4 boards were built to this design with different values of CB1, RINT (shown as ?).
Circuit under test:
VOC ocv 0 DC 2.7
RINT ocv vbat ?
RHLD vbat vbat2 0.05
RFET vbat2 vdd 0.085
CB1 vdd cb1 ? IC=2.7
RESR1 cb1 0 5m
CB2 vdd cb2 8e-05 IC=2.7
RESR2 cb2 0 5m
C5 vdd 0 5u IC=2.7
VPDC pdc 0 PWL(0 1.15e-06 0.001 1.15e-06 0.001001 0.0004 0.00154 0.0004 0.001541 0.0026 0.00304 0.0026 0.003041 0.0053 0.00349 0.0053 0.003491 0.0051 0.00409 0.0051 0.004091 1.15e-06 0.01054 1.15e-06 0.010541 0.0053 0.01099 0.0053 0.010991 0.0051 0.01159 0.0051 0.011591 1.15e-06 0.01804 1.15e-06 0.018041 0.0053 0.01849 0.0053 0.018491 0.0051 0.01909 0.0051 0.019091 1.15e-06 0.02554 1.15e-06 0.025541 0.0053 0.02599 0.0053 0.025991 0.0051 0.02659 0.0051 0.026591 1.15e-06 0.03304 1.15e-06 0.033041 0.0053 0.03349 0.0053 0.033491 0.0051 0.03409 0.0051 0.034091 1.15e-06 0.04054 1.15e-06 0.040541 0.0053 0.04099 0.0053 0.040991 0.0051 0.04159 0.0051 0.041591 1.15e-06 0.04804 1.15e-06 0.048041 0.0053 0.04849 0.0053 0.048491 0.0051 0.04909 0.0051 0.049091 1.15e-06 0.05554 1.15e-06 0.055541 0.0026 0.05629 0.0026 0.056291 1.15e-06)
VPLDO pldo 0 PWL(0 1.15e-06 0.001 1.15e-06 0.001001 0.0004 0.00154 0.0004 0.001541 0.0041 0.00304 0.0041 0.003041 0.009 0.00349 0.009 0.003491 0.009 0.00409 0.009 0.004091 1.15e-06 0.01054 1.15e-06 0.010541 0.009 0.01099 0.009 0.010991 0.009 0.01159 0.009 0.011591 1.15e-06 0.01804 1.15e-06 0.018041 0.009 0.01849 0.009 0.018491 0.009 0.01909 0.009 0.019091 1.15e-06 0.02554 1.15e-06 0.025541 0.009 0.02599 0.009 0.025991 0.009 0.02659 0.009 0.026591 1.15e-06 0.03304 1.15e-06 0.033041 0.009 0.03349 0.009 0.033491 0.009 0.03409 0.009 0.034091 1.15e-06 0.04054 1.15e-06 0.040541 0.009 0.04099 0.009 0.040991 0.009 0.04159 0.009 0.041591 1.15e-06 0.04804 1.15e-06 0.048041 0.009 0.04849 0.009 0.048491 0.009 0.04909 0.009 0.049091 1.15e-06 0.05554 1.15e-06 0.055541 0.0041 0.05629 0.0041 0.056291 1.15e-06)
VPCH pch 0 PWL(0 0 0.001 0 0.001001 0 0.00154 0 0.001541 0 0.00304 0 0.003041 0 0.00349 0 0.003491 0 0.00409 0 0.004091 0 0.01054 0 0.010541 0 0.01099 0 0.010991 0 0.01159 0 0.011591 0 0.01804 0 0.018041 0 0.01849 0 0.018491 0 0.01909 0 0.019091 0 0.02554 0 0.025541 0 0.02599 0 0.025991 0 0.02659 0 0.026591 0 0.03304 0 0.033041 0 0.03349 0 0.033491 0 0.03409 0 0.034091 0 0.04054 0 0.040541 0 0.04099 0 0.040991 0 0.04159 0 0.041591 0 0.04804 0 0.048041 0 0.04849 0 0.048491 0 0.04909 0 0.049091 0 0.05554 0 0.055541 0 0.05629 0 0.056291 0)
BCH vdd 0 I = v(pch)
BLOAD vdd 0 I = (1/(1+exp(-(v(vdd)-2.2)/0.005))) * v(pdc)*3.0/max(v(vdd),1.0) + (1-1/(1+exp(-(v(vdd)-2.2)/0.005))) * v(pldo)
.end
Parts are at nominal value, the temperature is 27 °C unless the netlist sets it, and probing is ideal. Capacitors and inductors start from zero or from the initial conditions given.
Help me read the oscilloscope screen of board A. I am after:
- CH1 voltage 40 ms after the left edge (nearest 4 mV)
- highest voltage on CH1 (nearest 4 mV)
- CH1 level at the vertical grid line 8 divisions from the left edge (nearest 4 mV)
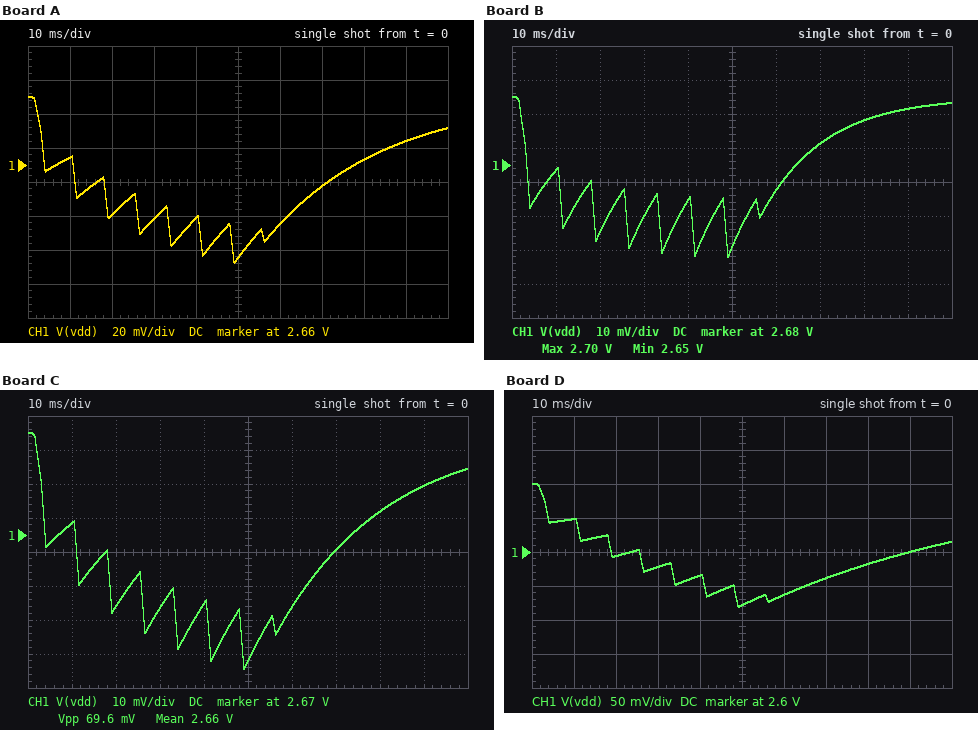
2.628 V
2.700 V
2.664 V
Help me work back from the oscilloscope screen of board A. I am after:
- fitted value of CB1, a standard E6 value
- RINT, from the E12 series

150 µF
120 Ω
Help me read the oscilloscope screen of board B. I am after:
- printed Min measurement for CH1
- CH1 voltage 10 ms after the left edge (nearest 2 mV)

2.65 V
2.678 V
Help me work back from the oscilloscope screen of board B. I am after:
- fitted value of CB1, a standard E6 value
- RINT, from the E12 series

220 µF
47 Ω
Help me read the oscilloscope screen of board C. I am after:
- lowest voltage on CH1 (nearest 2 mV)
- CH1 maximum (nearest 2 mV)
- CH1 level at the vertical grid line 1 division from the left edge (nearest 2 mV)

2.630 V
2.700 V
2.674 V
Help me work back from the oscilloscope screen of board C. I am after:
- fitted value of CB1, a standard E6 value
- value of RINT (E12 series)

220 µF
82 Ω
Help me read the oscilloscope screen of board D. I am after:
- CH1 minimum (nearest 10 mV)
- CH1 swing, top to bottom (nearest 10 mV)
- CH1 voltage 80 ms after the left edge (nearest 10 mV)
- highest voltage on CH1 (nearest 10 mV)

2.52 V
180 mV
2.58 V
2.70 V
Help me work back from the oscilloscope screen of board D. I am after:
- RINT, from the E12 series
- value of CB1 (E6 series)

330 Ω
100 µF
